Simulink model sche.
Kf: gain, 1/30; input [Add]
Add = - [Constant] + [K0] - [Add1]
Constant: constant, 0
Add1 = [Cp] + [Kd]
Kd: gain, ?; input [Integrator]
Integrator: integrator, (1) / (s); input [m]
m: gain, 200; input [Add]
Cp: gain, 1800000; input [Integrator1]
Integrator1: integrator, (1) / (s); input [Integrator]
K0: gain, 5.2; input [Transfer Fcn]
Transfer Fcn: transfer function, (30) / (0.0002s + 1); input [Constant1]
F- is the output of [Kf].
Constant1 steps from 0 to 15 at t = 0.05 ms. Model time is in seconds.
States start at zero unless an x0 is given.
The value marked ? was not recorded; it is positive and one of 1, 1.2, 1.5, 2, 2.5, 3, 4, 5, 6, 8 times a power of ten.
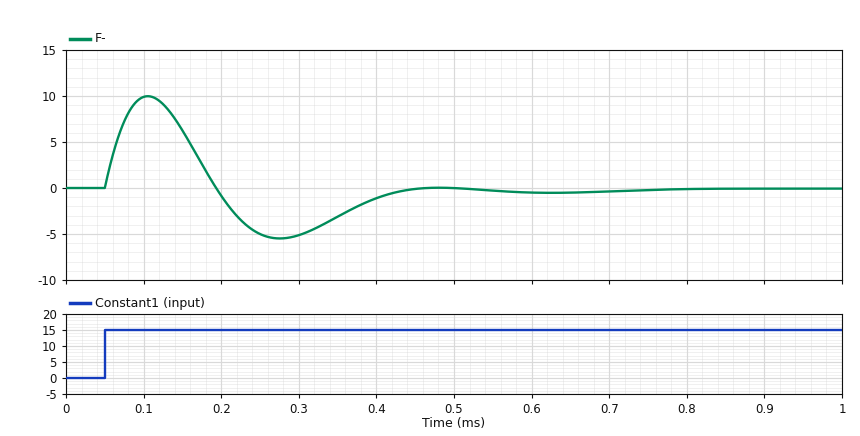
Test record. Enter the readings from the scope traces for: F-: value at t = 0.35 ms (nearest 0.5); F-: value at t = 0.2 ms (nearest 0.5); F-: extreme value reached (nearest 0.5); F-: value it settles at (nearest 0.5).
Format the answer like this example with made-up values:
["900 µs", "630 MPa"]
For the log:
["-3.0", "-1.0", "10.0", "0.0"]
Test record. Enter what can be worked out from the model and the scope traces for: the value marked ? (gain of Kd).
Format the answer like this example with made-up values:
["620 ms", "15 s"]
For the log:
["80"]
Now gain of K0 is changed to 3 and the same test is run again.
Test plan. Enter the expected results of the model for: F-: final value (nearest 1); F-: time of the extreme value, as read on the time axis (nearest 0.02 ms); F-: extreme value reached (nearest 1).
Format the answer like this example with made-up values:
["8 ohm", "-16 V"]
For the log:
["0", "0.10 ms", "6"]
